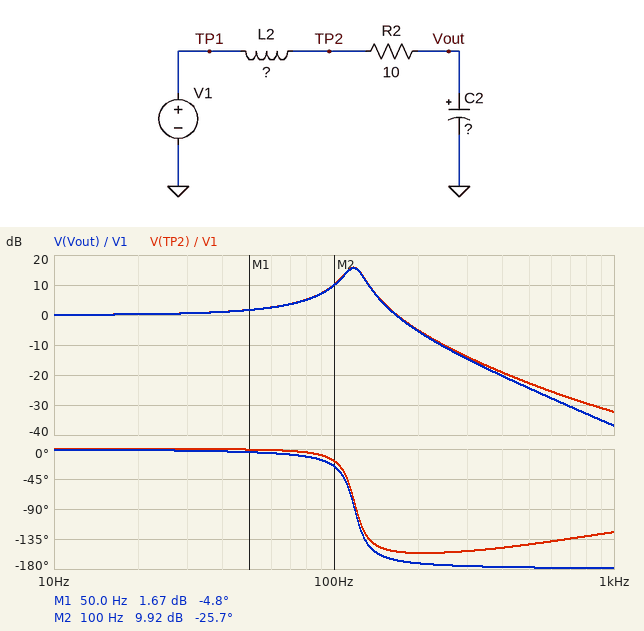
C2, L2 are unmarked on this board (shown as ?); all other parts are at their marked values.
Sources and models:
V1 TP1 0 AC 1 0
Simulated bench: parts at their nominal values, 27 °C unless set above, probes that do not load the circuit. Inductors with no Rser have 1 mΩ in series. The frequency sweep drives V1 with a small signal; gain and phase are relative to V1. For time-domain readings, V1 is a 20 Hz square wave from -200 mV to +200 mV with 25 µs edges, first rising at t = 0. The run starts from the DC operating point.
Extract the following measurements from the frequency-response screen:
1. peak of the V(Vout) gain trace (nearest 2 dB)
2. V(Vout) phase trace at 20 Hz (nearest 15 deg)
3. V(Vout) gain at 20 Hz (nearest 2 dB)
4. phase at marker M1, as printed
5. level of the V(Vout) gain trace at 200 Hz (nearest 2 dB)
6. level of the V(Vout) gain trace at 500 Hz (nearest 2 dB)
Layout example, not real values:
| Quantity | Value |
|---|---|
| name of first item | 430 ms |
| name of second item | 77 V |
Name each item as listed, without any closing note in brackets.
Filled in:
| Quantity | Value |
|---|---|
| peak of the V(Vout) gain trace | 16 dB |
| V(Vout) phase trace at 20 Hz | 0 deg |
| V(Vout) gain at 20 Hz | 0 dB |
| phase at marker M1, as printed | -4.8 deg |
| level of the V(Vout) gain trace at 200 Hz | -6 dB |
| level of the V(Vout) gain trace at 500 Hz | -24 dB |
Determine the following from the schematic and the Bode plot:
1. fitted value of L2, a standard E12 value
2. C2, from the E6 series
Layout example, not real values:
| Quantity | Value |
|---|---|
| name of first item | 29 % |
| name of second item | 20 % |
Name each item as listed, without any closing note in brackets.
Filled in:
| Quantity | Value |
|---|---|
| fitted value of L2, a standard E12 value | 82 mH |
| C2, from the E6 series | 22 µF |
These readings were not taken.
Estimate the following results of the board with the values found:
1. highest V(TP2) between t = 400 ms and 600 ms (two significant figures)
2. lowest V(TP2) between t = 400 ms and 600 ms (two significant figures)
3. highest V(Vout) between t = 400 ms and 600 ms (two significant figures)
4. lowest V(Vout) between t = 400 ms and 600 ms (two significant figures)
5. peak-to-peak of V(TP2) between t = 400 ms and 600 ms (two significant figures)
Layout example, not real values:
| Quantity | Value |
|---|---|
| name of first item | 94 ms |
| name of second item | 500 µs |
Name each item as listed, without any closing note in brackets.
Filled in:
| Quantity | Value |
|---|---|
| highest V(TP2) between t = 400 ms and 600 ms | 460 mV |
| lowest V(TP2) between t = 400 ms and 600 ms | -460 mV |
| highest V(Vout) between t = 400 ms and 600 ms | 460 mV |
| lowest V(Vout) between t = 400 ms and 600 ms | -460 mV |
| peak-to-peak of V(TP2) between t = 400 ms and 600 ms | 920 mV |
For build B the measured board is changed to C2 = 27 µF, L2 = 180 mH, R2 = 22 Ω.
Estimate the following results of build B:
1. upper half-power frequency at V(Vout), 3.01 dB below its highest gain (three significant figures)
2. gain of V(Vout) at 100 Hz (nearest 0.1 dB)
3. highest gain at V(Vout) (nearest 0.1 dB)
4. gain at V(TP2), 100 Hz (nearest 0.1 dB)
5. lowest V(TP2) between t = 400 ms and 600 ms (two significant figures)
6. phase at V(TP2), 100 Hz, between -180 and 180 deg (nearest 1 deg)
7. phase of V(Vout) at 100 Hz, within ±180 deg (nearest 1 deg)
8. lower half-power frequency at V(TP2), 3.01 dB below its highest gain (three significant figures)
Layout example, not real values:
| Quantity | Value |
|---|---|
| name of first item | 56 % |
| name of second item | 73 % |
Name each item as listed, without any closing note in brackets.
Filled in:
| Quantity | Value |
|---|---|
| upper half-power frequency at V(Vout), 3.01 dB below its highest gain | 80.1 Hz |
| gain of V(Vout) at 100 Hz | 0.1 dB |
| highest gain at V(Vout) | 11.5 dB |
| gain at V(TP2), 100 Hz | 0.6 dB |
| lowest V(TP2) between t = 400 ms and 600 ms | -460 mV |
| phase at V(TP2), 100 Hz, between -180 and 180 deg | -137 deg |
| phase of V(Vout) at 100 Hz, within ±180 deg | -158 deg |
| lower half-power frequency at V(TP2), 3.01 dB below its highest gain | 60.5 Hz |
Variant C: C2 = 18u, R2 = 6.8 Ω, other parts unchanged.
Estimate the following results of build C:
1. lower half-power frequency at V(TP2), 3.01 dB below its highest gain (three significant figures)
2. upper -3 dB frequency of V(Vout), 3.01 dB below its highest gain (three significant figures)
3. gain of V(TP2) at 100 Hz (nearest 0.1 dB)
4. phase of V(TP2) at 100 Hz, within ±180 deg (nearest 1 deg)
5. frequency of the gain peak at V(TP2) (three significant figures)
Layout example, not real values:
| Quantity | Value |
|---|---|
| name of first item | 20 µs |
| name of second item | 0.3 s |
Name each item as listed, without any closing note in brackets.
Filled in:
| Quantity | Value |
|---|---|
| lower half-power frequency at V(TP2), 3.01 dB below its highest gain | 124 Hz |
| upper -3 dB frequency of V(Vout), 3.01 dB below its highest gain | 137 Hz |
| gain of V(TP2) at 100 Hz | 7.5 dB |
| phase of V(TP2) at 100 Hz, within ±180 deg | -6 deg |
| frequency of the gain peak at V(TP2) | 131 Hz |
